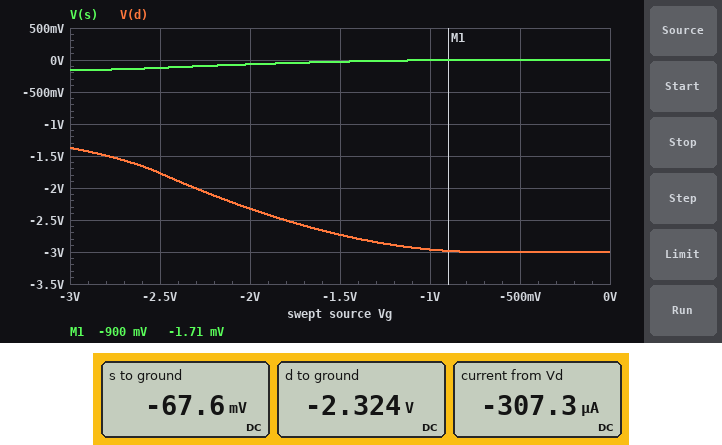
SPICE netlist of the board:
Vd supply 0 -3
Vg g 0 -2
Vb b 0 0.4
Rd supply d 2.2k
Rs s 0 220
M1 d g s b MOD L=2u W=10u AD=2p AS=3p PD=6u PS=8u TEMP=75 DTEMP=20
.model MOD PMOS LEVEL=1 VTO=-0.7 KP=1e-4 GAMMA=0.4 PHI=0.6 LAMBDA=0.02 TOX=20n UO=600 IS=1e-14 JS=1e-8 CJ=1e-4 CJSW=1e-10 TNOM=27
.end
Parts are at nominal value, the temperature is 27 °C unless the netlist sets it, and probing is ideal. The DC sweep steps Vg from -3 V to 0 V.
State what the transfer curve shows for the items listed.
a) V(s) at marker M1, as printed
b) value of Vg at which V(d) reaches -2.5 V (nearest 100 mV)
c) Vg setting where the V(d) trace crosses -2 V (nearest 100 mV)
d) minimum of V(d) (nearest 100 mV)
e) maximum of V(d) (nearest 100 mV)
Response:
-1.71 mV
-1.8 V
-2.3 V
-3.0 V
-1.4 V
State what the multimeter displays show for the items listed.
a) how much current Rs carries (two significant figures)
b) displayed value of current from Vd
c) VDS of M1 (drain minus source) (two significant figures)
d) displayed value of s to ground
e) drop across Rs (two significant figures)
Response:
310 µA
-307.3 µA
-2.3 V
-67.6 mV
68 mV
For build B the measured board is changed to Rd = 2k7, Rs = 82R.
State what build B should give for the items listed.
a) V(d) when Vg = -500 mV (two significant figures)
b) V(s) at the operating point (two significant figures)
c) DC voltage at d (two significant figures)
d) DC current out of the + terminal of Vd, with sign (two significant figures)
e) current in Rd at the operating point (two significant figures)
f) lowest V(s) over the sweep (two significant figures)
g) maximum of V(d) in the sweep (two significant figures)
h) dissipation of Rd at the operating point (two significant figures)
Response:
-3.0 V
-27 mV
-2.1 V
-330 µA
330 µA
-58 mV
-1.1 V
300 µW
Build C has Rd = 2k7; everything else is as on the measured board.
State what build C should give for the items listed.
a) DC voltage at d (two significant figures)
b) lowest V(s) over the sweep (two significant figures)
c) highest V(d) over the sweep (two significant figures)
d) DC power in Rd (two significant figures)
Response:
-2.2 V
-150 mV
-1.2 V
250 µW
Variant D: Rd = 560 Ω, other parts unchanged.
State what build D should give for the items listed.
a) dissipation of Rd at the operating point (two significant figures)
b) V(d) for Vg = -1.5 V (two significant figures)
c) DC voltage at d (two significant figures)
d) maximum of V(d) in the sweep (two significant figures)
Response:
54 µW
-2.9 V
-2.8 V
-2.5 V
